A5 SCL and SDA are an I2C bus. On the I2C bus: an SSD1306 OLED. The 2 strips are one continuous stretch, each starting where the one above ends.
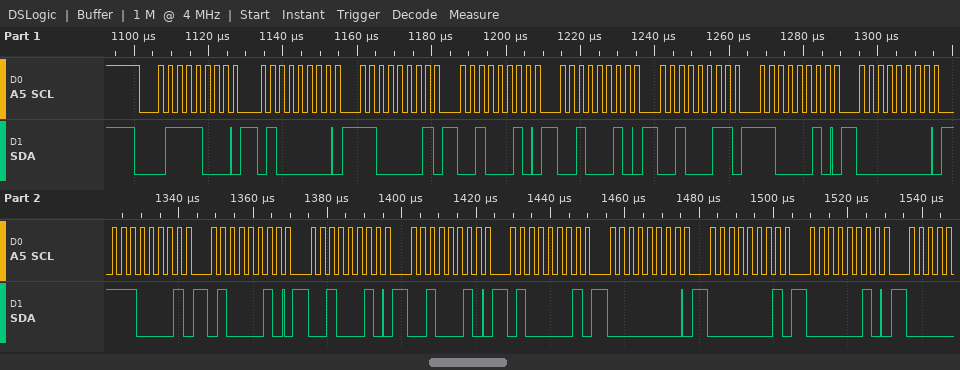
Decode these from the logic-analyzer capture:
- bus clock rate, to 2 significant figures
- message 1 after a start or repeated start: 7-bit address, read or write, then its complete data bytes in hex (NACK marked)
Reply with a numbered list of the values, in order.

1. 400 kHz
2. 0x3C write: 40 C1 22 22 23 C2 00 E1 42 22 22 41 00 01 02
